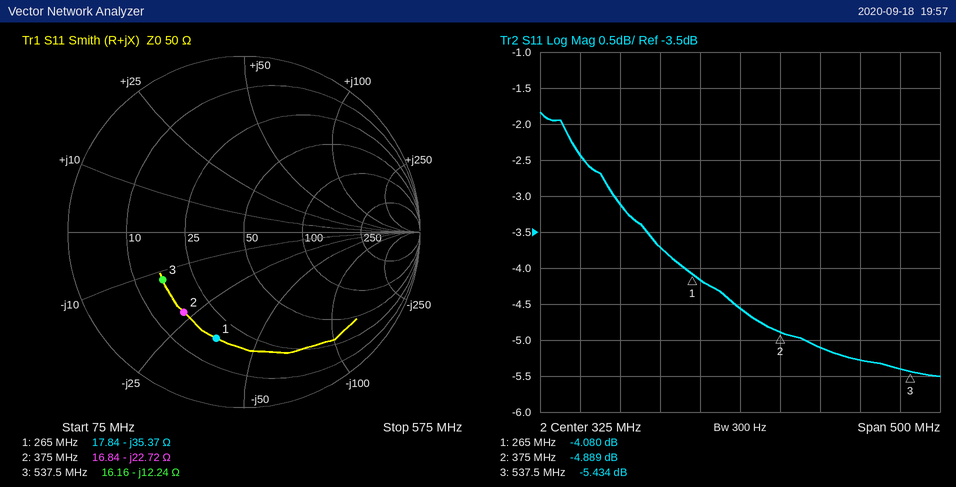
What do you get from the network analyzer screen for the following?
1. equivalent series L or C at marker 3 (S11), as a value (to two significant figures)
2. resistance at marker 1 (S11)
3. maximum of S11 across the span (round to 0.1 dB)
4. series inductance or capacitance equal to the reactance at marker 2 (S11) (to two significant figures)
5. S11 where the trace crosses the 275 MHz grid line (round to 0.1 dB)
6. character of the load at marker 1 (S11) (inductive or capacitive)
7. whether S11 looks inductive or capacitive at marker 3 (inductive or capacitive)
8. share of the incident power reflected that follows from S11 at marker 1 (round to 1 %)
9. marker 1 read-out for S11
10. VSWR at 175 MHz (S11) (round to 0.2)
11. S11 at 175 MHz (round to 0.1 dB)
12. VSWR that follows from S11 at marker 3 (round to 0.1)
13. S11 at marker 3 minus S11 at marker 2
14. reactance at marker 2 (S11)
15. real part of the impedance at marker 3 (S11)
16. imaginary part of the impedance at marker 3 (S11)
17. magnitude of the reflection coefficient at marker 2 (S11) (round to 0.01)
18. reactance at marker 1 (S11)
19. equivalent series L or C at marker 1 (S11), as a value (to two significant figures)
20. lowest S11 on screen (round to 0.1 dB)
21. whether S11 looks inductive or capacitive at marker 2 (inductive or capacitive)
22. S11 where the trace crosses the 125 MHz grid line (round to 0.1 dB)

24 pF
17.84 Ω
-1.8 dB
19 pF
-4.2 dB
capacitive
capacitive
39 %
-4.080 dB
5.6
-3.1 dB
3.3
-0.545 dB
-22.72 Ω
16.16 Ω
-12.24 Ω
0.57
-35.37 Ω
17 pF
-5.5 dB
capacitive
-2.4 dB
